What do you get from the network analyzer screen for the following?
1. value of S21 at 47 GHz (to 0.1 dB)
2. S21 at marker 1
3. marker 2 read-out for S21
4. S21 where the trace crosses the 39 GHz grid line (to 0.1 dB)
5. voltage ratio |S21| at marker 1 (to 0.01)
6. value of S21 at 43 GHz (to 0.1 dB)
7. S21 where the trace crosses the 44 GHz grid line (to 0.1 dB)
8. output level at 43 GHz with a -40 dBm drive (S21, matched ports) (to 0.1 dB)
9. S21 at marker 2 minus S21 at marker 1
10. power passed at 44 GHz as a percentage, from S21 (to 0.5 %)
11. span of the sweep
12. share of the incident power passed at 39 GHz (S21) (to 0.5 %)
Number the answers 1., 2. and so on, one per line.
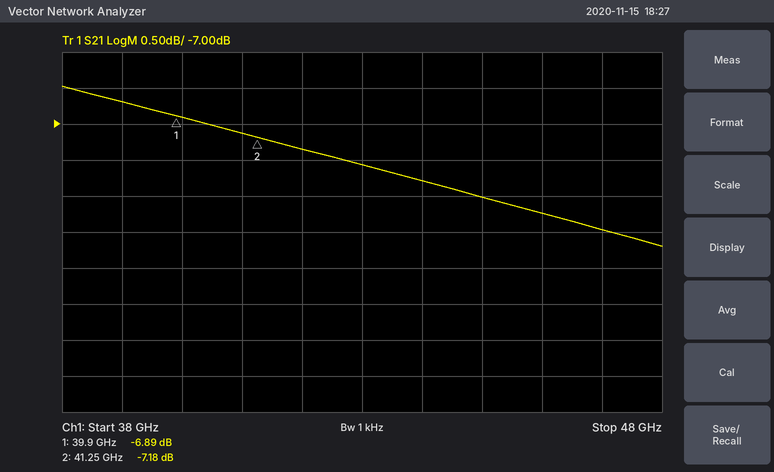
1. -8.5 dB
2. -6.89 dB
3. -7.18 dB
4. -6.7 dB
5. 0.45
6. -7.6 dB
7. -7.8 dB
8. -47.6 dBm
9. -0.29 dB
10. 16.5 %
11. 10 GHz
12. 21.5 %
